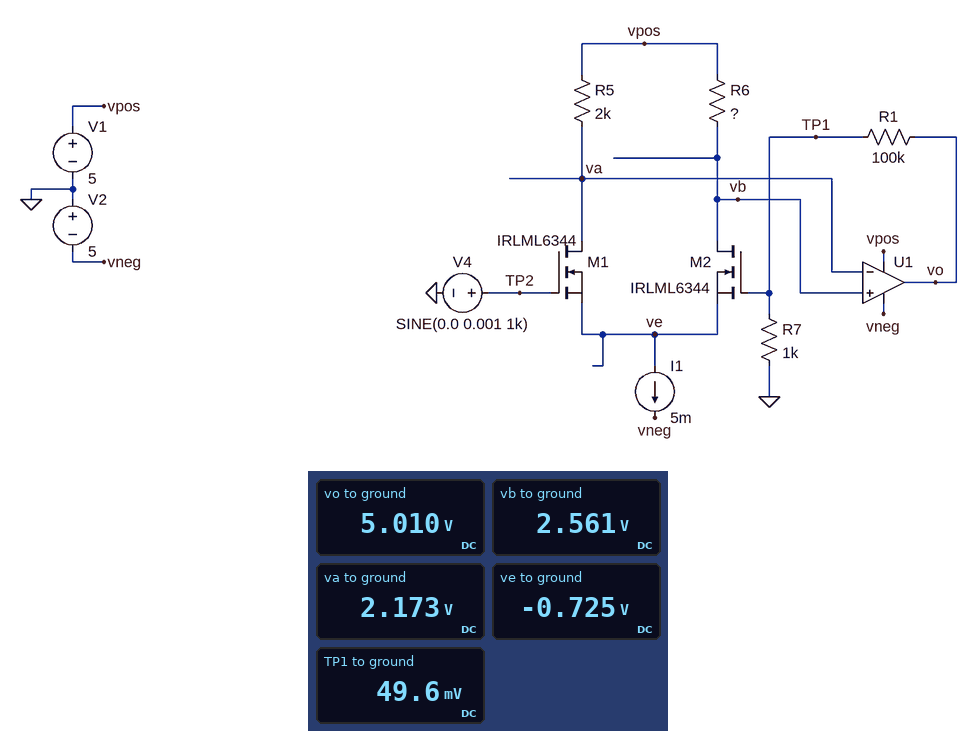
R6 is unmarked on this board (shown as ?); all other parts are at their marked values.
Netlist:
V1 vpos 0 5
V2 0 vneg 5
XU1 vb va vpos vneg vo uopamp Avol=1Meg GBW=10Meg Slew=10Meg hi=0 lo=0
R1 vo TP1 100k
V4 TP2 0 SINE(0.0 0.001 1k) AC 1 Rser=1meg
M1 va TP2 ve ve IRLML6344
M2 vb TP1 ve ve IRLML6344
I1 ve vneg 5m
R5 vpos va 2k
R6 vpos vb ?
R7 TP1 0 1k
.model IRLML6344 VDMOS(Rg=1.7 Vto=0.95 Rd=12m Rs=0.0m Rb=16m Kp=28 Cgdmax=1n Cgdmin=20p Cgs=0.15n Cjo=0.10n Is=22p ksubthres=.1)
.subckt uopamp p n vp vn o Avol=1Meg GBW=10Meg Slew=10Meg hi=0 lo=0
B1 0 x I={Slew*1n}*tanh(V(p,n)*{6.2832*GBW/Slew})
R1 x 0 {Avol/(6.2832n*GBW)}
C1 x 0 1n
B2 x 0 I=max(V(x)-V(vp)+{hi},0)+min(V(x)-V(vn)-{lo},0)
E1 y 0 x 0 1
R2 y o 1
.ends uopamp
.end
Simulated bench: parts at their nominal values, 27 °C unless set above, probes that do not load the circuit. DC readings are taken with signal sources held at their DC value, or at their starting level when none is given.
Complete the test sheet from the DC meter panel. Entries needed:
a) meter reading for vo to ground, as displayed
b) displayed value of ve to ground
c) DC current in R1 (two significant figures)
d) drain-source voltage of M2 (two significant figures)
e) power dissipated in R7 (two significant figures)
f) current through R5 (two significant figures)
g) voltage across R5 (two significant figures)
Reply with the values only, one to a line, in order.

5.010 V
-0.725 V
50 µA
3.3 V
2.5 µW
1.4 mA
2.8 V
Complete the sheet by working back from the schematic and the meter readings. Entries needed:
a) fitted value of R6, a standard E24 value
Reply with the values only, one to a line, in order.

680 Ω
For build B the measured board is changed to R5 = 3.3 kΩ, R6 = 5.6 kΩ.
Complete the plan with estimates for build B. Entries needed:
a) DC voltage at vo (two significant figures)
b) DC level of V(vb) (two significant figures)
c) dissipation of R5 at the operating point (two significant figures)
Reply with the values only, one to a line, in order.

-5.0 V
-5.4 V
33 mW
